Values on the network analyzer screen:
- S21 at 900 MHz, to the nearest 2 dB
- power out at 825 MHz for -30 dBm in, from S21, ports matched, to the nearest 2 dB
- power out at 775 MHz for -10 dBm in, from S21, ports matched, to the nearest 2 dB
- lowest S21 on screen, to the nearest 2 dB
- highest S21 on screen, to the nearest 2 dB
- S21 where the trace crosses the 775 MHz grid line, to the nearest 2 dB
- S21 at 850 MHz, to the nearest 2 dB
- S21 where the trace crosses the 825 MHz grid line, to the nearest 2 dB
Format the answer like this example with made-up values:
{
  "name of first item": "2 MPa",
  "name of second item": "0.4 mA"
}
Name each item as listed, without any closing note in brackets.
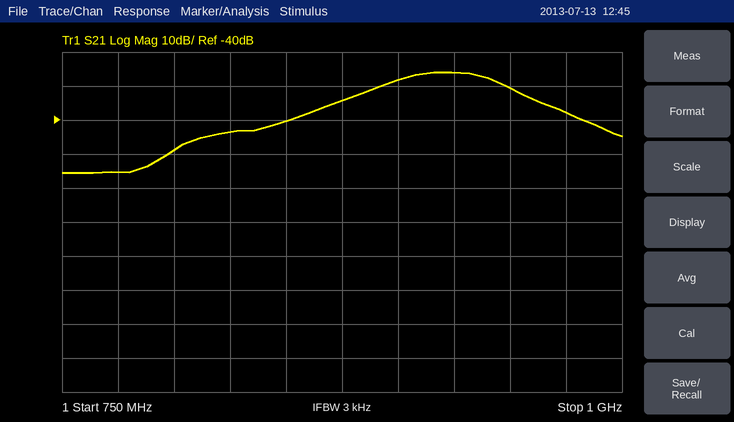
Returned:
{
  "S21 at 900 MHz, to the nearest 2 dB": "-28 dB",
  "power out at 825 MHz for -30 dBm in, from S21, ports matched, to the nearest 2 dB": "-74 dBm",
  "power out at 775 MHz for -10 dBm in, from S21, ports matched, to the nearest 2 dB": "-66 dBm",
  "lowest S21 on screen, to the nearest 2 dB": "-56 dB",
  "highest S21 on screen, to the nearest 2 dB": "-26 dB",
  "S21 where the trace crosses the 775 MHz grid line, to the nearest 2 dB": "-56 dB",
  "S21 at 850 MHz, to the nearest 2 dB": "-40 dB",
  "S21 where the trace crosses the 825 MHz grid line, to the nearest 2 dB": "-44 dB"
}
